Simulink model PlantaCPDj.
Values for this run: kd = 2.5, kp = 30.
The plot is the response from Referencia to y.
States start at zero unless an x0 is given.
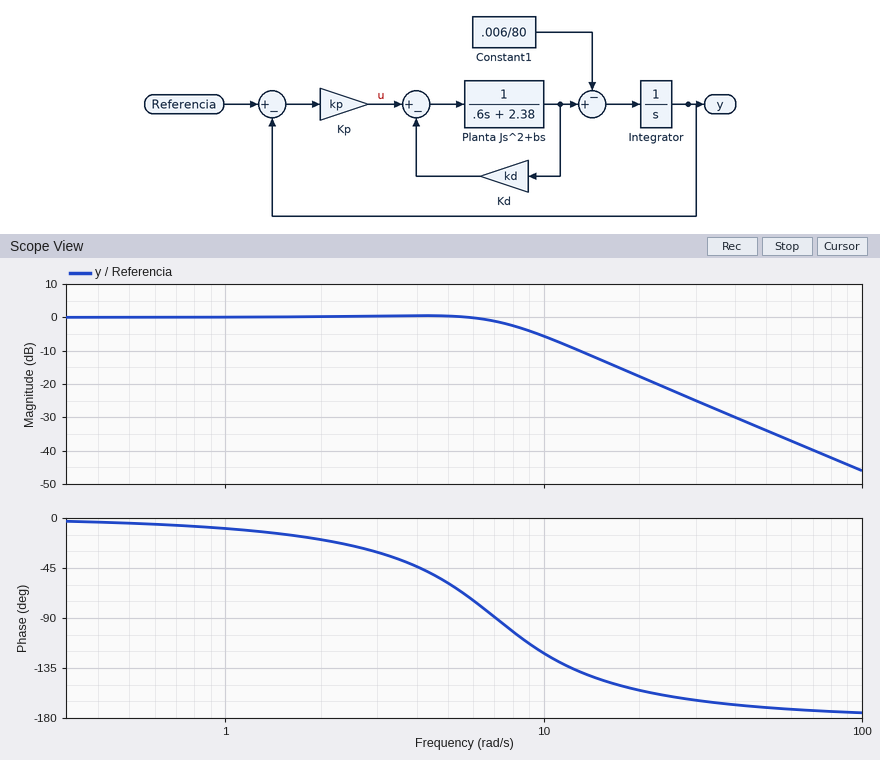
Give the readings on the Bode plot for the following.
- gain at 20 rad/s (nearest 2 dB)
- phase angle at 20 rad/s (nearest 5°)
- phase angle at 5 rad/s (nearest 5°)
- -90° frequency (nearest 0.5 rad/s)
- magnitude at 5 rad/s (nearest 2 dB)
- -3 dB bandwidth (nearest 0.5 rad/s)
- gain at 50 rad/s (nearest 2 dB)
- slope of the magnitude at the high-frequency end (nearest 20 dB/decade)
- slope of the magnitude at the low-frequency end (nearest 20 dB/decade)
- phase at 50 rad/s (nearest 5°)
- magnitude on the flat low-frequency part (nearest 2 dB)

-18 dB
-155°
-60°
7.0 rad/s
0 dB
8.5 rad/s
-34 dB
-40 dB/decade
0 dB/decade
-170°
0 dB
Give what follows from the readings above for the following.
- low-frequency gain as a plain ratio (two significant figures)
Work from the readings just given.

1.0
